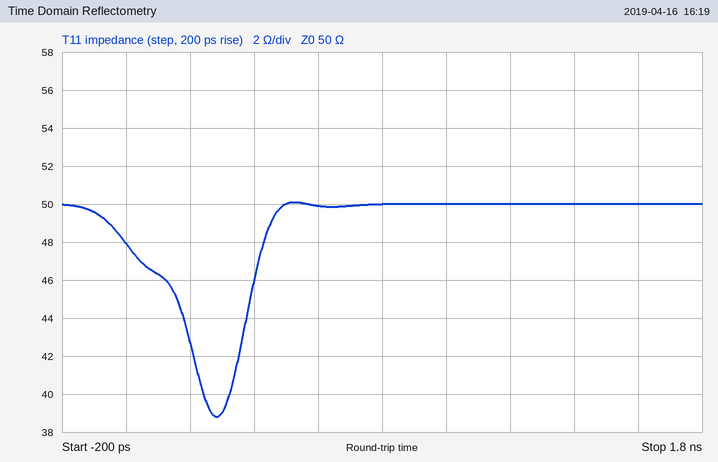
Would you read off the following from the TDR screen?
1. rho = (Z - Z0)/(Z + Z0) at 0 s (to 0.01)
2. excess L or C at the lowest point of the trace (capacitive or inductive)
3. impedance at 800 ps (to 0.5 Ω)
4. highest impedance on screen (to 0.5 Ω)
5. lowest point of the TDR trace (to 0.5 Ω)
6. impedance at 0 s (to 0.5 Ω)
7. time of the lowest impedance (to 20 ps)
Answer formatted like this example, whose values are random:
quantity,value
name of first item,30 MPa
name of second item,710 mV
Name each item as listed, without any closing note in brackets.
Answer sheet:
quantity,value
rho = (Z - Z0)/(Z + Z0) at 0 s,-0.02
excess L or C at the lowest point of the trace,capacitive
impedance at 800 ps,50.0 Ω
highest impedance on screen,50.0 Ω
lowest point of the TDR trace,39.0 Ω
impedance at 0 s,48.0 Ω
time of the lowest impedance,280 ps
